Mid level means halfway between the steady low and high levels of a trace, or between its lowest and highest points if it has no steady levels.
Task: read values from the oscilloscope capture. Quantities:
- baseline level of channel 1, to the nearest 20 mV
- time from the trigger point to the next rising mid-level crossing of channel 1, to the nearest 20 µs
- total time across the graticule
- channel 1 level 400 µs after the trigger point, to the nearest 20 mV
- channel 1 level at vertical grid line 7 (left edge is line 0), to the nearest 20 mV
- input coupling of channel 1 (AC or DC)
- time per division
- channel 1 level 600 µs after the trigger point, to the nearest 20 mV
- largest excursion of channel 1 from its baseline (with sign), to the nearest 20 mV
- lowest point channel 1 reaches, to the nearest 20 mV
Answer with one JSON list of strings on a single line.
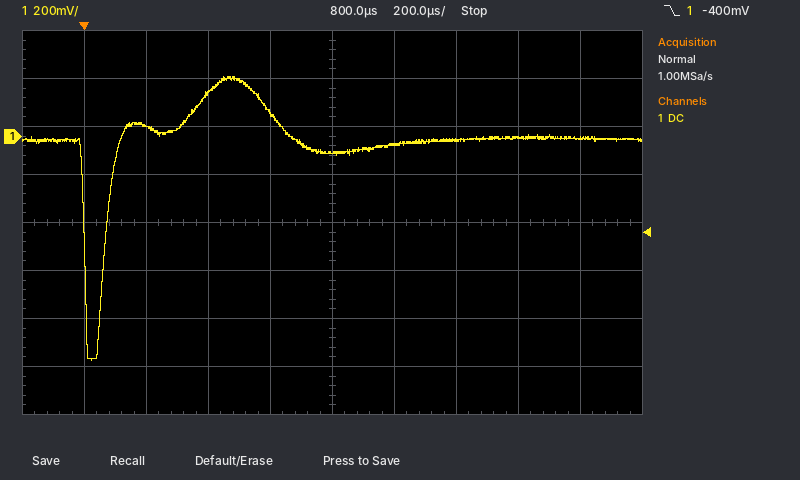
["-20 mV", "80 µs", "2 ms", "180 mV", "-20 mV", "DC", "200 µs", "100 mV", "-920 mV", "-940 mV"]
